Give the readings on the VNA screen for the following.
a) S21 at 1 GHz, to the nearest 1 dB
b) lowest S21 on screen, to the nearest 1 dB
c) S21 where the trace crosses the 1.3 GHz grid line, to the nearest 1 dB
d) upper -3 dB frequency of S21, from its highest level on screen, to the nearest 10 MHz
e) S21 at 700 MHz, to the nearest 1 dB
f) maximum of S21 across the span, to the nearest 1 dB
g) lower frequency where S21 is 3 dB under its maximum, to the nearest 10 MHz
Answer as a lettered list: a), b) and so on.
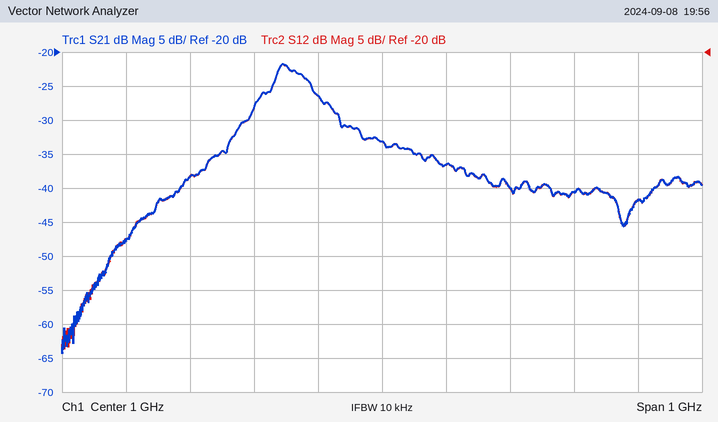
a) -33 dB
b) -64 dB
c) -41 dB
d) 890 MHz
e) -38 dB
f) -22 dB
g) 830 MHz
